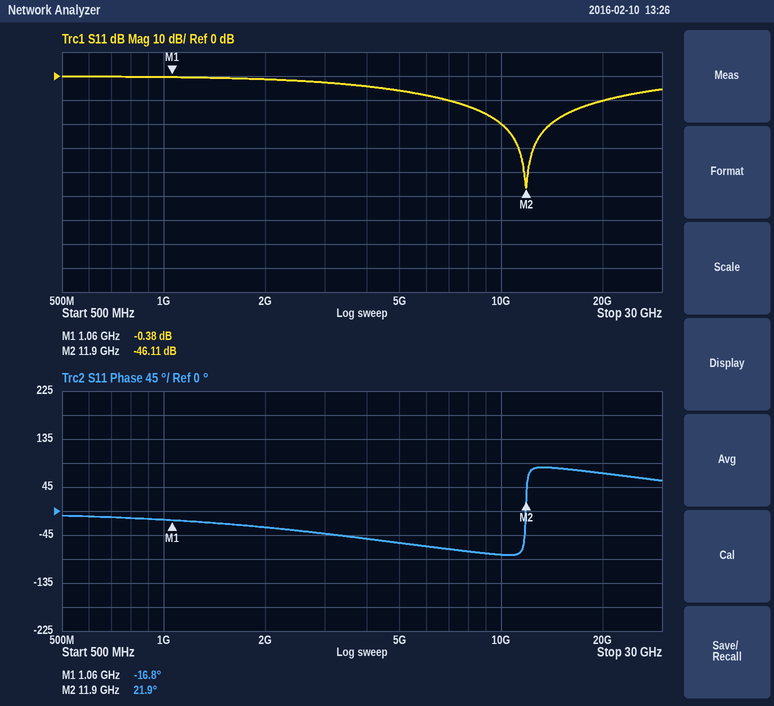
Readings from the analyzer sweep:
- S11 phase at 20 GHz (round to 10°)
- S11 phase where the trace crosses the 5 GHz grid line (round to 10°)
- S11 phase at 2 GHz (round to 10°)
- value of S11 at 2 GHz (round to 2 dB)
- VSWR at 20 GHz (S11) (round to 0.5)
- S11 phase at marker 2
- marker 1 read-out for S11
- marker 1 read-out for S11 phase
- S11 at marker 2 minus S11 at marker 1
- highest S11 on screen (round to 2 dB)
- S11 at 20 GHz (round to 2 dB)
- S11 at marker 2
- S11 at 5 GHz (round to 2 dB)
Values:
70°
-60°
-30°
-2 dB
2.0
21.9°
-0.38 dB
-16.8°
-45.73 dB
0 dB
-10 dB
-46.11 dB
-6 dB
